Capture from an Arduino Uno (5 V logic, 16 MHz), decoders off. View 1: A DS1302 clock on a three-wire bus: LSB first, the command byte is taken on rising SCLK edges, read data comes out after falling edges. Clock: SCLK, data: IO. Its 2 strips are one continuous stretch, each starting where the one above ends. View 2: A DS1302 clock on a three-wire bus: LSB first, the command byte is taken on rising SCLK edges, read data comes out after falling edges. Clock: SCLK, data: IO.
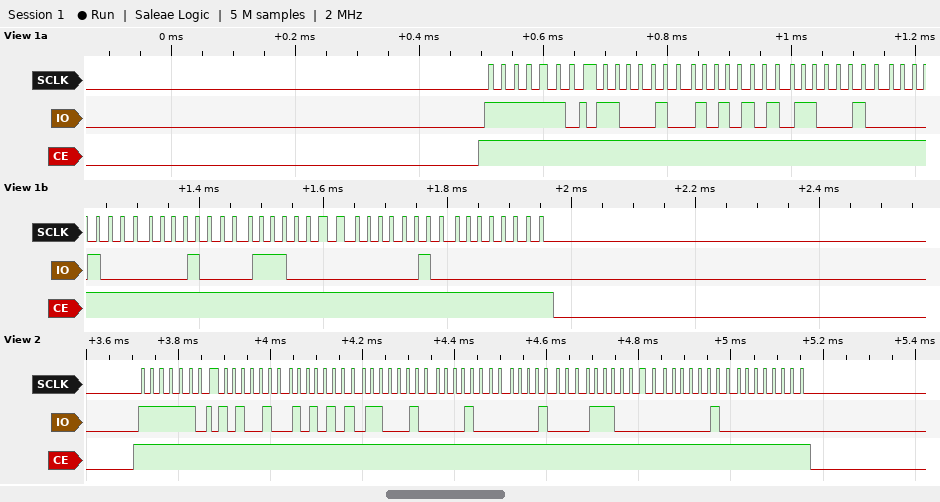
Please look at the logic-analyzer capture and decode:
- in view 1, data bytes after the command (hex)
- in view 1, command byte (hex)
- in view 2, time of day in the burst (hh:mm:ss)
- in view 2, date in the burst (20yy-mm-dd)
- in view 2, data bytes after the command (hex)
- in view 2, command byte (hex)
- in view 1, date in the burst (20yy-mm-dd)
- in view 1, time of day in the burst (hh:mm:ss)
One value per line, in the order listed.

23 55 23 08 08 07 20 00
0xBF
23:55:25
2020-08-08
25 55 23 08 08 07 20 00
0xBF
2020-08-08
23:55:23
